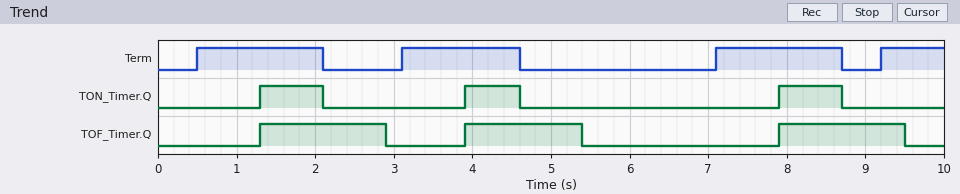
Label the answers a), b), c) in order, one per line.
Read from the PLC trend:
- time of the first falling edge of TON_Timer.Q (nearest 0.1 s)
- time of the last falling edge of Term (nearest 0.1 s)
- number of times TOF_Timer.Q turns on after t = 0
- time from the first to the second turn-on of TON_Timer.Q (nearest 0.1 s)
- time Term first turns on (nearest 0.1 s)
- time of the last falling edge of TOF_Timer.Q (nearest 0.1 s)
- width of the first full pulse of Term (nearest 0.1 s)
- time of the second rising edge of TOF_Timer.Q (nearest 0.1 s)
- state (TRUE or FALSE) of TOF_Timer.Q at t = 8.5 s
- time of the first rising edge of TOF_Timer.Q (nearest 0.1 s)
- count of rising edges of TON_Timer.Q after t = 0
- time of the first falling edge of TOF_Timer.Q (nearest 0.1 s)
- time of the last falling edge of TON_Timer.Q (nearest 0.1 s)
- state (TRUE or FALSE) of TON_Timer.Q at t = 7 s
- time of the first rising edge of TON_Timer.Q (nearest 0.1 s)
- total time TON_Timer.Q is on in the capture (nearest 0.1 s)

a) 2.1 s
b) 8.7 s
c) 3
d) 2.6 s
e) 0.5 s
f) 9.5 s
g) 1.6 s
h) 3.9 s
i) TRUE
j) 1.3 s
k) 3
l) 2.9 s
m) 8.7 s
n) FALSE
o) 1.3 s
p) 2.3 s
